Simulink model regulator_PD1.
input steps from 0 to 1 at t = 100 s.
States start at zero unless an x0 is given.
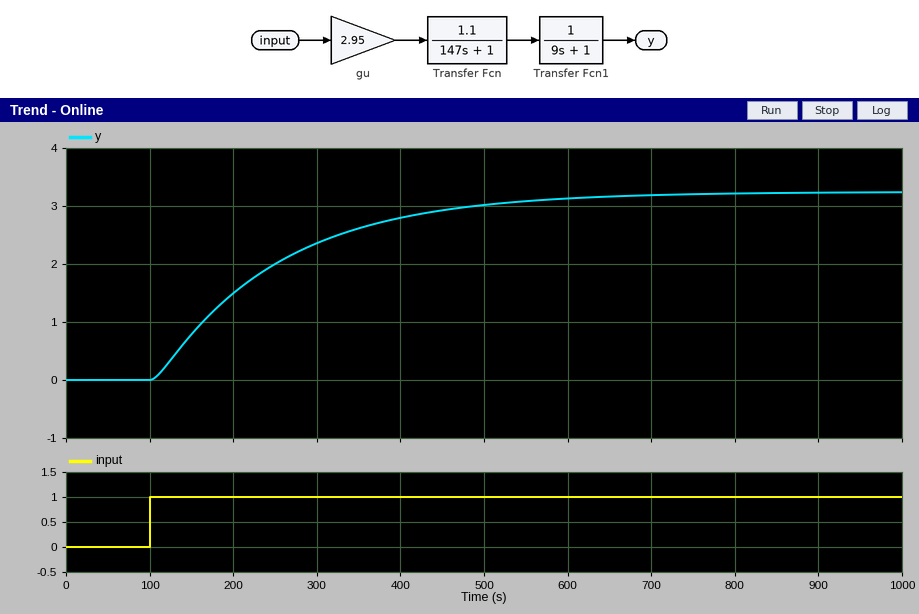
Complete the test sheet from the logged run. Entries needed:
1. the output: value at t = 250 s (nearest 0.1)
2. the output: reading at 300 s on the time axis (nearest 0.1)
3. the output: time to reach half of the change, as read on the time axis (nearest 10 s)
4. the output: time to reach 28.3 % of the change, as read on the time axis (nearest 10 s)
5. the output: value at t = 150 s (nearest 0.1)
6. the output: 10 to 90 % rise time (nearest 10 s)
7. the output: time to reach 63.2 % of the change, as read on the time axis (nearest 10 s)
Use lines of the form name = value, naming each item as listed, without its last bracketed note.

the output: value at t = 250 s = 2.0
the output: reading at 300 s on the time axis = 2.4
the output: time to reach half of the change, as read on the time axis = 210 s
the output: time to reach 28.3 % of the change, as read on the time axis = 160 s
the output: value at t = 150 s = 0.8
the output: 10 to 90 % rise time = 320 s
the output: time to reach 63.2 % of the change, as read on the time axis = 260 s
